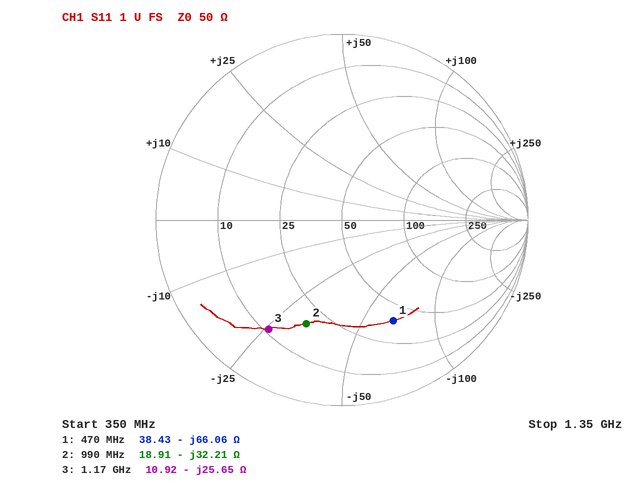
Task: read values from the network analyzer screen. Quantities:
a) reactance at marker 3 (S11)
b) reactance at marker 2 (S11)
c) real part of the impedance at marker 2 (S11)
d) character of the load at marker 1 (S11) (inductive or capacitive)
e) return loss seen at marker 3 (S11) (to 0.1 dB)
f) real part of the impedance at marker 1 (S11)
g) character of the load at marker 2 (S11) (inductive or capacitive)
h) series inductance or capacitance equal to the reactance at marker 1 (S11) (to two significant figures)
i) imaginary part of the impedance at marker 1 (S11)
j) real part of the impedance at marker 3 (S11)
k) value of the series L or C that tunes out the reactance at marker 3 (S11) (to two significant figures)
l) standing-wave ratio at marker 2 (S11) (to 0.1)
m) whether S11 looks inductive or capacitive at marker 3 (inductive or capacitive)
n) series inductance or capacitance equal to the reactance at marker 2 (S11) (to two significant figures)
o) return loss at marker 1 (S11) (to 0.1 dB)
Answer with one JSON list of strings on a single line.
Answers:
["-25.65 Ω", "-32.21 Ω", "18.91 Ω", "capacitive", "3.0 dB", "38.43 Ω", "capacitive", "5.1 pF", "-66.06 Ω", "10.92 Ω", "3.5 nH", "3.9", "capacitive", "5.0 pF", "4.3 dB"]
